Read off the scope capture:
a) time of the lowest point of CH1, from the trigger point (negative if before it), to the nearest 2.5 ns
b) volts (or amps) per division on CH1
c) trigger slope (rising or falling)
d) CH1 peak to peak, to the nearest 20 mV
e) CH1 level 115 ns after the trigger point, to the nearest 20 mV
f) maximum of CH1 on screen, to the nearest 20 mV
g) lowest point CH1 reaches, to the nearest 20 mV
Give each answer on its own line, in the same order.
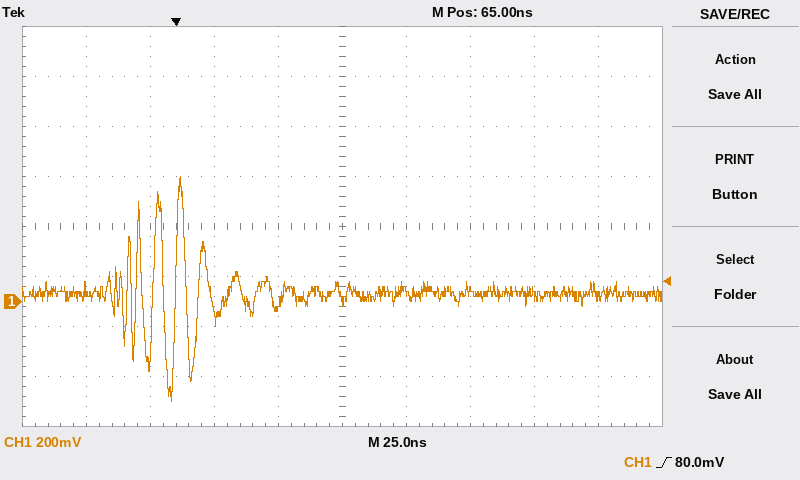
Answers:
-2.5 ns
200 mV
rising
900 mV
40 mV
500 mV
-400 mV
